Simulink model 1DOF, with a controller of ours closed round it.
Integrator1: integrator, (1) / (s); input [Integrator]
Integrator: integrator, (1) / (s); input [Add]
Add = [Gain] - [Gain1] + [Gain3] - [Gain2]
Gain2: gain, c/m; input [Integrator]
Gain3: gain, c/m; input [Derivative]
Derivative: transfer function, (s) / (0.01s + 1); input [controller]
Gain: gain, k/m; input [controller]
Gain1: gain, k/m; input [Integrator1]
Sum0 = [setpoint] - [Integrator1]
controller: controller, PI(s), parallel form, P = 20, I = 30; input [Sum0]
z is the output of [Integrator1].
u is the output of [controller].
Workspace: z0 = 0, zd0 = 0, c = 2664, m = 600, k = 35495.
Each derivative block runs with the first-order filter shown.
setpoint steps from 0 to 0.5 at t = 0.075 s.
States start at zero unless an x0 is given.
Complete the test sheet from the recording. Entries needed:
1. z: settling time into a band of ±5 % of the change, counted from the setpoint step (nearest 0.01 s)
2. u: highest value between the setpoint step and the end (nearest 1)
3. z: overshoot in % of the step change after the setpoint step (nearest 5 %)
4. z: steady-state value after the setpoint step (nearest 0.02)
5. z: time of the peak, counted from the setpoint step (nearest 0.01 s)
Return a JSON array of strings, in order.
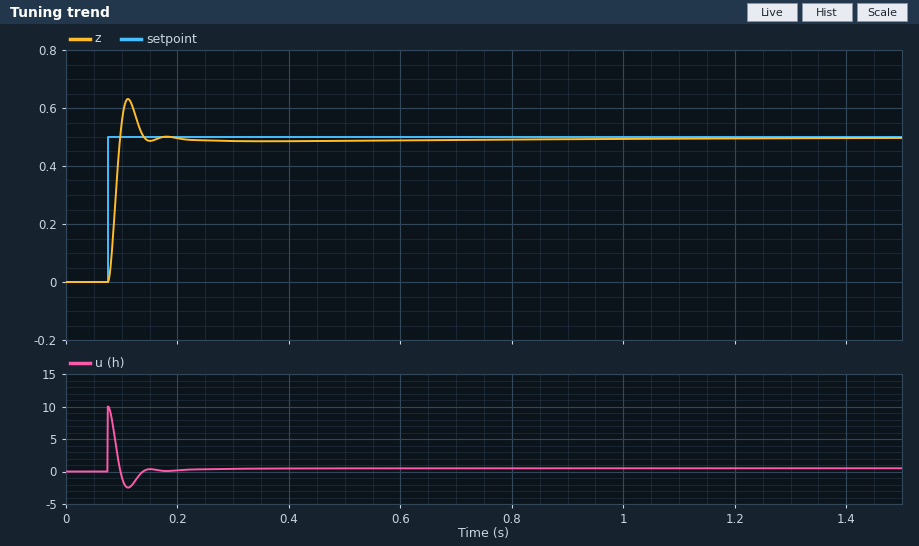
["0.06 s", "10", "25 %", "0.50", "0.04 s"]
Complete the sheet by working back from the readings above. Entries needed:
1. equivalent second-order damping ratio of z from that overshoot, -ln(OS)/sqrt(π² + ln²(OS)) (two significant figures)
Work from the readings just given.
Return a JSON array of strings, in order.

["0.40"]
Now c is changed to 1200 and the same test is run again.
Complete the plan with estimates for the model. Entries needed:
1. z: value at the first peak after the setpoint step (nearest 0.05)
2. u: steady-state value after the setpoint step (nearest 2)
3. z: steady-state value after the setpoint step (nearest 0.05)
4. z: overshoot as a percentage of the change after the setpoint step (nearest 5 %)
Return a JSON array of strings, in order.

["0.70", "0", "0.50", "35 %"]
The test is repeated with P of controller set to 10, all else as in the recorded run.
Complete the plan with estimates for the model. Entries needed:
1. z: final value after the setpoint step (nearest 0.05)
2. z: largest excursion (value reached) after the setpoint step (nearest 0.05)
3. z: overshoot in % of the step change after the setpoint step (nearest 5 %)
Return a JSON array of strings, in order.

["0.50", "0.60", "20 %"]
